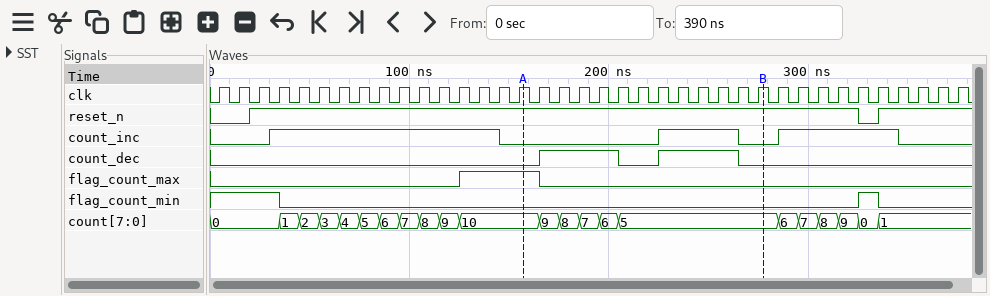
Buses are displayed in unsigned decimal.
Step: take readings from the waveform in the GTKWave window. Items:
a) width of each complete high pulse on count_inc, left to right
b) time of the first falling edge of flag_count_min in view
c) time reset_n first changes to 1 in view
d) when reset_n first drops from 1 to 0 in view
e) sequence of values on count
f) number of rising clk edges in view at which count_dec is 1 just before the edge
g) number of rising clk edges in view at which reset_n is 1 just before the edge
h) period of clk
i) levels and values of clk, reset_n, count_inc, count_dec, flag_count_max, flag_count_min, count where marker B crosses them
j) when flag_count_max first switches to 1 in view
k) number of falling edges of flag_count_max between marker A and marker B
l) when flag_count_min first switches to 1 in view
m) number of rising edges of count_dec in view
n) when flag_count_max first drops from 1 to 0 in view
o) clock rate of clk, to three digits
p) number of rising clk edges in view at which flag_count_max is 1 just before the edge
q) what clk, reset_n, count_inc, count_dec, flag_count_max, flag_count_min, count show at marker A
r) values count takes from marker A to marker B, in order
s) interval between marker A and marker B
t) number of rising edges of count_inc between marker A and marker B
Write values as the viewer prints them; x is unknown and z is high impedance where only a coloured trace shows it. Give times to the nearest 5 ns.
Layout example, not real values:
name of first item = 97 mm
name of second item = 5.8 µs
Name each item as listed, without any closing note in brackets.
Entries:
width of each complete high pulse on count_inc, left to right = 115 ns, 40 ns, 60 ns
time of the first falling edge of flag_count_min in view = 35 ns
time reset_n first changes to 1 in view = 20 ns
when reset_n first drops from 1 to 0 in view = 325 ns
sequence of values on count = 0, 1, 2, 3, 4, 5, 6, 7, 8, 9, 10, 9, 8, 7, 6, 5, 6, 7, 8, 9, 0, 1
number of rising clk edges in view at which count_dec is 1 just before the edge = 8
number of rising clk edges in view at which reset_n is 1 just before the edge = 35
period of clk = 10 ns
levels and values of clk, reset_n, count_inc, count_dec, flag_count_max, flag_count_min, count where marker B crosses them = clk=1, reset_n=1, count_inc=0, count_dec=0, flag_count_max=0, flag_count_min=0, count=5
when flag_count_max first switches to 1 in view = 125 ns
number of falling edges of flag_count_max between marker A and marker B = 1
when flag_count_min first switches to 1 in view = 325 ns
number of rising edges of count_dec in view = 2
when flag_count_max first drops from 1 to 0 in view = 165 ns
clock rate of clk, to three digits = 100 MHz
number of rising clk edges in view at which flag_count_max is 1 just before the edge = 4
what clk, reset_n, count_inc, count_dec, flag_count_max, flag_count_min, count show at marker A = clk=1, reset_n=1, count_inc=0, count_dec=0, flag_count_max=1, flag_count_min=0, count=10
values count takes from marker A to marker B, in order = 10, 9, 8, 7, 6, 5
interval between marker A and marker B = 120 ns
number of rising edges of count_inc between marker A and marker B = 1
